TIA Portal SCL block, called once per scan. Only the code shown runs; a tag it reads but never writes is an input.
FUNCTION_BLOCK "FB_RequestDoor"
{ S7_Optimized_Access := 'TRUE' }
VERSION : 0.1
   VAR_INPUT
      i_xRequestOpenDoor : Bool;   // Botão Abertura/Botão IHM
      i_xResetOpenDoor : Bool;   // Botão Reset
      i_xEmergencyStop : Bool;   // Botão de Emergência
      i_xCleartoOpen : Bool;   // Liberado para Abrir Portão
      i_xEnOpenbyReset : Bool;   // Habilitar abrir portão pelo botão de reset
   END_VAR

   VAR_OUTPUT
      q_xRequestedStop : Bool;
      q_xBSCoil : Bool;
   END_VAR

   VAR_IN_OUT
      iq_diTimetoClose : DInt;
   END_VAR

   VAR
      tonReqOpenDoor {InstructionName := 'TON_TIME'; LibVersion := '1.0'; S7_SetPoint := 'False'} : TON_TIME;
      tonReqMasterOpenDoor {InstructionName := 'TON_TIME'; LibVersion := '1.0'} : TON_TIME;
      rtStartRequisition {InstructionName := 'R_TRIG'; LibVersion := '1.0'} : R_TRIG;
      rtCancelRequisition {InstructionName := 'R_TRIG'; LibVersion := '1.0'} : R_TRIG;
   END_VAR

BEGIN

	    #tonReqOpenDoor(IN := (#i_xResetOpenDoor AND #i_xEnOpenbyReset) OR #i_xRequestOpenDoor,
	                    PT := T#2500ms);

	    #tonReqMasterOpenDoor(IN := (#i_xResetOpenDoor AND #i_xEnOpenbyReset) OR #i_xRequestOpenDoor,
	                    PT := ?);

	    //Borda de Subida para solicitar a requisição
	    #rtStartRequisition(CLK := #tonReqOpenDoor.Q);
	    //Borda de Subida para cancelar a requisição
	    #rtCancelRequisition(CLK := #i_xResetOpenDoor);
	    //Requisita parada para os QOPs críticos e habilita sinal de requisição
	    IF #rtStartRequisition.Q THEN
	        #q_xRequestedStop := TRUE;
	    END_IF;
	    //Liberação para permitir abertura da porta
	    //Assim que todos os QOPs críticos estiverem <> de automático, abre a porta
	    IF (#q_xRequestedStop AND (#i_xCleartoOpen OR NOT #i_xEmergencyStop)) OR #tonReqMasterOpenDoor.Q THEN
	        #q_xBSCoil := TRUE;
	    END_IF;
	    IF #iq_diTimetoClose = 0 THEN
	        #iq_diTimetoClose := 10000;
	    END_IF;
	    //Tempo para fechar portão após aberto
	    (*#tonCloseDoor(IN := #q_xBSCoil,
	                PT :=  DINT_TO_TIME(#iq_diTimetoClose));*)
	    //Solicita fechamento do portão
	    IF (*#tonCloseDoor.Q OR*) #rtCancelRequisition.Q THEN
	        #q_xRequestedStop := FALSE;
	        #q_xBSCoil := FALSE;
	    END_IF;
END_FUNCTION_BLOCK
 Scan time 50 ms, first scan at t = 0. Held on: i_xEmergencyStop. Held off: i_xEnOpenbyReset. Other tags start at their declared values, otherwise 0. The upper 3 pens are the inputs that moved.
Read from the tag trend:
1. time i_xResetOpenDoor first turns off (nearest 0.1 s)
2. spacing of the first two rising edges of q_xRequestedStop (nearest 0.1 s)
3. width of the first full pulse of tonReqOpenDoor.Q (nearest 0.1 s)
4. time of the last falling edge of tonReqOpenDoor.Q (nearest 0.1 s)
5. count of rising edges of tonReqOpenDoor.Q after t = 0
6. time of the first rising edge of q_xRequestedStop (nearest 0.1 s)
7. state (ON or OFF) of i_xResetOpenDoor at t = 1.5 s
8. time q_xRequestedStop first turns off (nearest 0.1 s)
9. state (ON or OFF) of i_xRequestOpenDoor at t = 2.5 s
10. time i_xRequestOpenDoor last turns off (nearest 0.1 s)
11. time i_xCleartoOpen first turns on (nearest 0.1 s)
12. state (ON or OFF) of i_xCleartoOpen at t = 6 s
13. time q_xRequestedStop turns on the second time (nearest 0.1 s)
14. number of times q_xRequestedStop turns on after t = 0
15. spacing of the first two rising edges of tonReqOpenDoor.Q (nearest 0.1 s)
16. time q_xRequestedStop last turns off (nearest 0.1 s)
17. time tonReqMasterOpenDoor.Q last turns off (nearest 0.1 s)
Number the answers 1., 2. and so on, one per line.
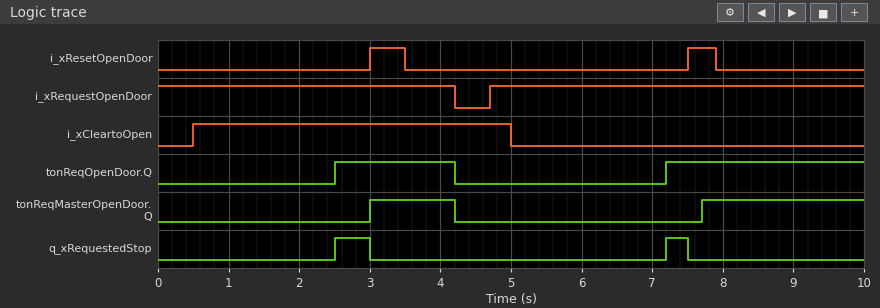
1. 3.5 s
2. 4.7 s
3. 1.7 s
4. 4.2 s
5. 2
6. 2.5 s
7. OFF
8. 3.0 s
9. ON
10. 4.2 s
11. 0.5 s
12. OFF
13. 7.2 s
14. 2
15. 4.7 s
16. 7.5 s
17. 4.2 s
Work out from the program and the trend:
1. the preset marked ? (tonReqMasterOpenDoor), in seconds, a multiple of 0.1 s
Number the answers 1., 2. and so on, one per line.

1. 3.0 s
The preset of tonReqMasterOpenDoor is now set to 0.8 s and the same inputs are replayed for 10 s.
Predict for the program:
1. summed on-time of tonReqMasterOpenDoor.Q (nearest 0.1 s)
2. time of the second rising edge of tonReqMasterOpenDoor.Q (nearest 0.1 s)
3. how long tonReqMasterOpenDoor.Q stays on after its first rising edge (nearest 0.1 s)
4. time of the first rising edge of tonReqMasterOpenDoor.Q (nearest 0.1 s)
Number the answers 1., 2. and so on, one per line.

1. 7.9 s
2. 5.5 s
3. 3.4 s
4. 0.8 s
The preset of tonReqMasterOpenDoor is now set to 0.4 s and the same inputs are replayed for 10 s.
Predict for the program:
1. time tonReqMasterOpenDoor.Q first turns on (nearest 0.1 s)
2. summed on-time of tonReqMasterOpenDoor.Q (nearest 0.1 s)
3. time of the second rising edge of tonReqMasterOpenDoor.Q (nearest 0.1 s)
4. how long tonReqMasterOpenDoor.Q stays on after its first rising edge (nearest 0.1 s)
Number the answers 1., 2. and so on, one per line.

1. 0.4 s
2. 8.7 s
3. 5.1 s
4. 3.8 s
